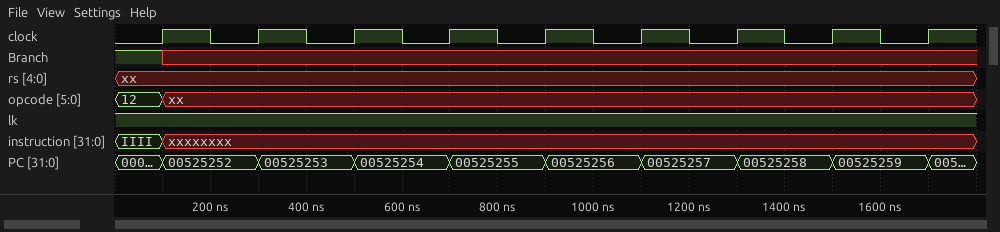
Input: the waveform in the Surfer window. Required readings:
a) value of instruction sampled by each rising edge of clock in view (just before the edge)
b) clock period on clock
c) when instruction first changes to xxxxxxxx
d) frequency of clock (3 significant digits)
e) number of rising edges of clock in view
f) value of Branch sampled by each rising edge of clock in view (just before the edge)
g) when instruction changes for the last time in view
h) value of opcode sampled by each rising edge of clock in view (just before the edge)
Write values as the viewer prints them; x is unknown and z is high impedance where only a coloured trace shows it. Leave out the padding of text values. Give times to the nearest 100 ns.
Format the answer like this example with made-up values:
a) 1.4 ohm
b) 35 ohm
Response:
a) IIII, xxxxxxxx, xxxxxxxx, xxxxxxxx, xxxxxxxx, xxxxxxxx, xxxxxxxx, xxxxxxxx, xxxxxxxx
b) 200 ns
c) 100 ns
d) 5.00 MHz
e) 9
f) 1 x x x x x x x x
g) 100 ns
h) 12, xx, xx, xx, xx, xx, xx, xx, xx
